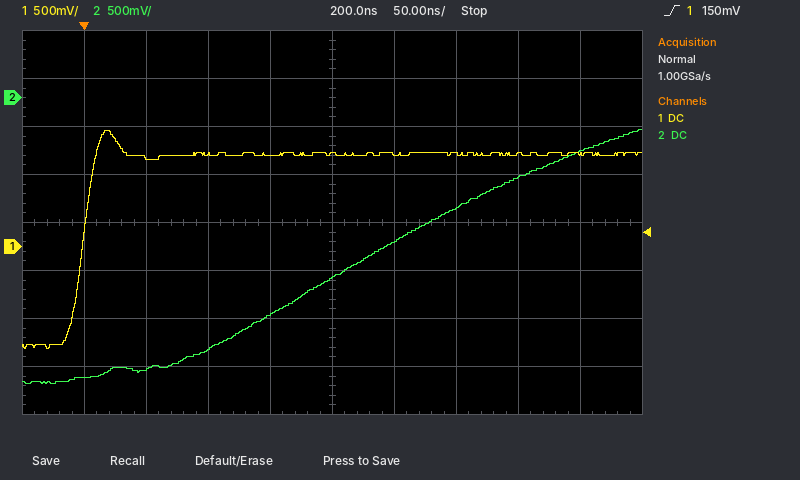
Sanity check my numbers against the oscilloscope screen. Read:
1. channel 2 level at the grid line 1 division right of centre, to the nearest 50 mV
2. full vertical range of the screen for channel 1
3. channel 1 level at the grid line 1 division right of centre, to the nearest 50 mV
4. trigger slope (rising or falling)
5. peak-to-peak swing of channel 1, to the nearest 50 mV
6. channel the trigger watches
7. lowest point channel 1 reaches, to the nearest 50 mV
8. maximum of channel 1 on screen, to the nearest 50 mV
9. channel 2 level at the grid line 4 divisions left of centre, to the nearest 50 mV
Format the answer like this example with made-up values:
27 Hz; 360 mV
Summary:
-1.50 V; 4 V; 950 mV; rising; 2.25 V; channel 1; -1.05 V; 1.20 V; -2.90 V
